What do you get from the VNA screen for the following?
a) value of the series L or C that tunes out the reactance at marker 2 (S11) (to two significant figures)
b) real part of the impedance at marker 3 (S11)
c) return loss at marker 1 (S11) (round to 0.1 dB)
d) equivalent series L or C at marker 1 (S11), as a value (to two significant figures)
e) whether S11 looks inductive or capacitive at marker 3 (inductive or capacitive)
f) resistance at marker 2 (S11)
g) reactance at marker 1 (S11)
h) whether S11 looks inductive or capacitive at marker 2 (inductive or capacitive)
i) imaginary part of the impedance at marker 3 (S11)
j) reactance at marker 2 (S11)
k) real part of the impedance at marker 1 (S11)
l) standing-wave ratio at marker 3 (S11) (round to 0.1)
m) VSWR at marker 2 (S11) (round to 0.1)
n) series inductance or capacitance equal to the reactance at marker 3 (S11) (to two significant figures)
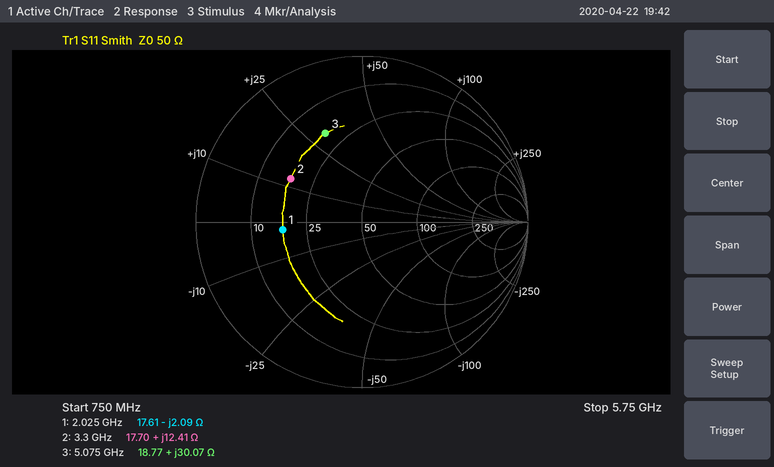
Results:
3.9 pF
18.77 Ω
6.4 dB
38 pF
inductive
17.70 Ω
-2.09 Ω
inductive
+30.07 Ω
+12.41 Ω
17.61 Ω
3.7
3.0
940 pH
